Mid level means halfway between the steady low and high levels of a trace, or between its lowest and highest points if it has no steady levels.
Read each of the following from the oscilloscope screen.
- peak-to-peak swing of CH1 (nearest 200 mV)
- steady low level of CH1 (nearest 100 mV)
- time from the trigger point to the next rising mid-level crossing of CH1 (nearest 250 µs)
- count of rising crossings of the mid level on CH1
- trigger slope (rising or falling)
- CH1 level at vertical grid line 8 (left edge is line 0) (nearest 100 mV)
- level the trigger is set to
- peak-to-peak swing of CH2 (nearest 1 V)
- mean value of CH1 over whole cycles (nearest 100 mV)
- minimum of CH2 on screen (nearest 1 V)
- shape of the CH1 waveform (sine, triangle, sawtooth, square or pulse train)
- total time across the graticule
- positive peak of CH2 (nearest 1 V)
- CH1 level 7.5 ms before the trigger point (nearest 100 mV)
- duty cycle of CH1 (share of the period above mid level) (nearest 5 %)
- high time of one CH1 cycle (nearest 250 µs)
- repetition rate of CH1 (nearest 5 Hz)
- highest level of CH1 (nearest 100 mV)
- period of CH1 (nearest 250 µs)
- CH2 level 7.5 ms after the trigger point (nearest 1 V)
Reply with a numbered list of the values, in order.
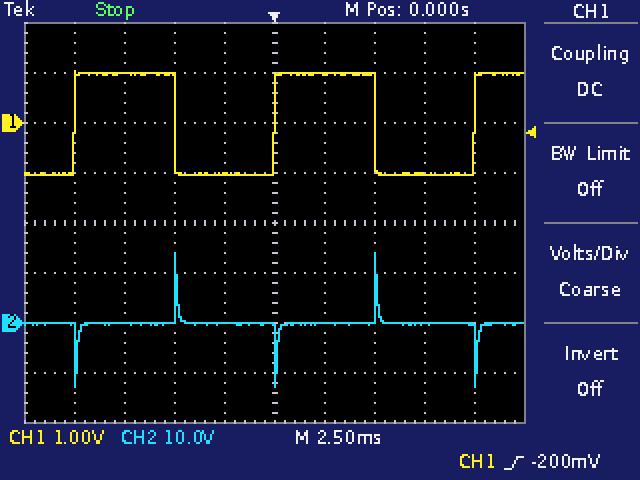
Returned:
1. 2.0 V
2. -1.0 V
3. 10.00 ms
4. 3
5. rising
6. -1.0 V
7. -200 mV
8. 27 V
9. 0.0 V
10. -13 V
11. square
12. 25 ms
13. 14 V
14. 1.0 V
15. 50 %
16. 5.00 ms
17. 100 Hz
18. 1.0 V
19. 10.00 ms
20. 0 V
